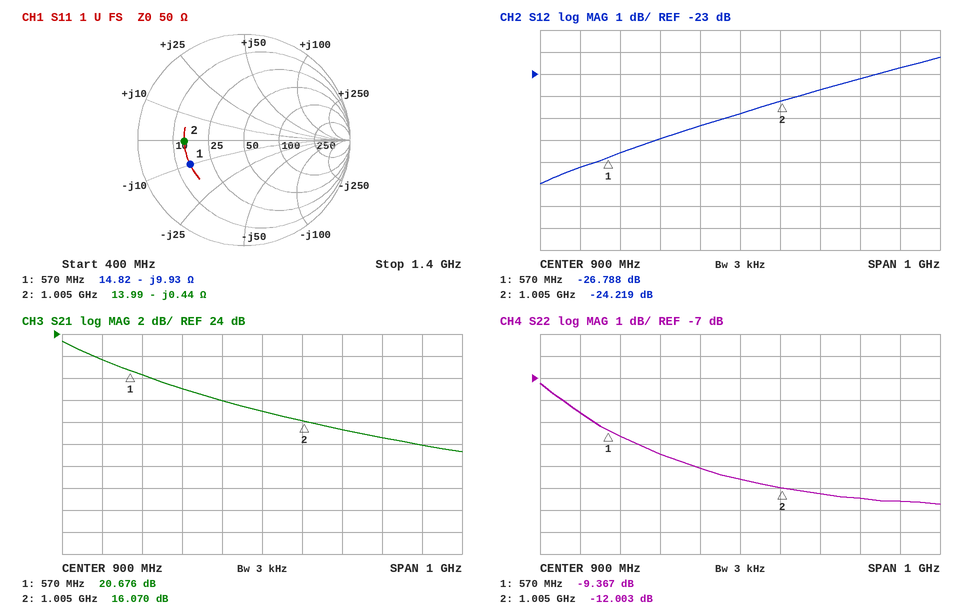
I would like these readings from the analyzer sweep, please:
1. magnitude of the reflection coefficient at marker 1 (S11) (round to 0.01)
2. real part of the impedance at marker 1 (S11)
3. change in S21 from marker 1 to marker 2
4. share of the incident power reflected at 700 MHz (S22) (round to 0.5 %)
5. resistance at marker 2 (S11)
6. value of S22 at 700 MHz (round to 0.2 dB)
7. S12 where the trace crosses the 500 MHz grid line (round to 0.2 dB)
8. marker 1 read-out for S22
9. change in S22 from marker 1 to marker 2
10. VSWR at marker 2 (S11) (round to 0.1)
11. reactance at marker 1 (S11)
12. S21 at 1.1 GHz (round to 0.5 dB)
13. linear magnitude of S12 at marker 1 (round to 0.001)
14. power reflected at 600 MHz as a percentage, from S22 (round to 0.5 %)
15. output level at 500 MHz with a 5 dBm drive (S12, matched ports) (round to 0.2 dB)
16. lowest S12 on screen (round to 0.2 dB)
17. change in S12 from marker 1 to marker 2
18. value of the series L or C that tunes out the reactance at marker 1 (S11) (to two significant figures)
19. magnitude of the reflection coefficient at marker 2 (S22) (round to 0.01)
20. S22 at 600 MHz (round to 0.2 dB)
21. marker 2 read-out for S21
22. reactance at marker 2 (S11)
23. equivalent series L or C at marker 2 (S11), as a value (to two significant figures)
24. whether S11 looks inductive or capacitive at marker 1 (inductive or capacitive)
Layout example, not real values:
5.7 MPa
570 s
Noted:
0.56
14.82 Ω
-4.606 dB
9.0 %
13.99 Ω
-10.4 dB
-27.2 dB
-9.367 dB
-2.636 dB
3.6
-9.93 Ω
15.5 dB
0.046
11.0 %
-22.2 dBm
-28.0 dB
2.569 dB
2.8 nH
0.25
-9.6 dB
16.070 dB
-0.44 Ω
360 pF
capacitive
